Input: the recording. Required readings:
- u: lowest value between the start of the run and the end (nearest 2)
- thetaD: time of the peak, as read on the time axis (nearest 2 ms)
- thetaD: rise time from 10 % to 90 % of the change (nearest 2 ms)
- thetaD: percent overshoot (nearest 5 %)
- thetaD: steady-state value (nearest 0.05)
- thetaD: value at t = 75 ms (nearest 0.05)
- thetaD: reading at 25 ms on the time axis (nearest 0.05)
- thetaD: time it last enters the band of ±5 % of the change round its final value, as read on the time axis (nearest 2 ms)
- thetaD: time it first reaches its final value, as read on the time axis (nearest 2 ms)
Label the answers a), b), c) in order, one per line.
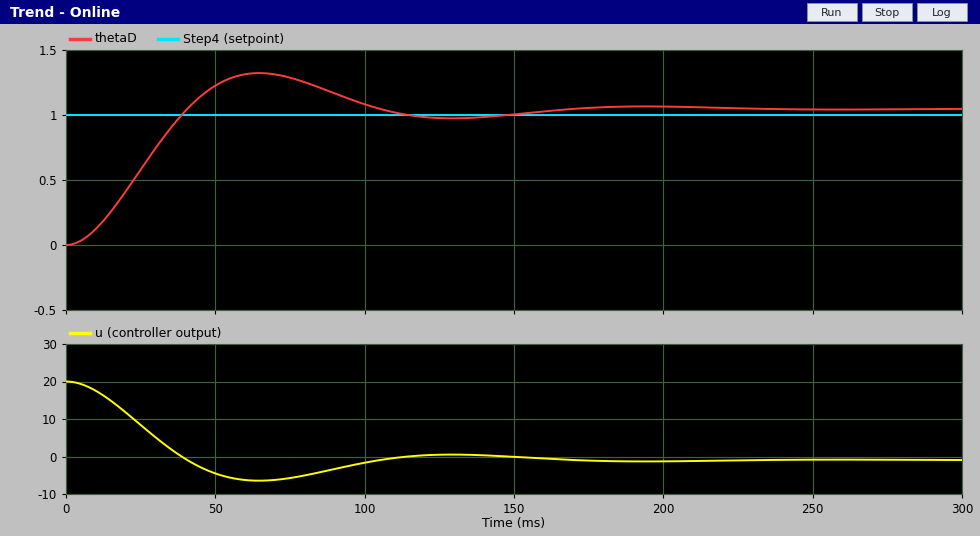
a) -6
b) 64 ms
c) 28 ms
d) 25 %
e) 1.05
f) 1.30
g) 0.60
h) 146 ms
i) 40 ms
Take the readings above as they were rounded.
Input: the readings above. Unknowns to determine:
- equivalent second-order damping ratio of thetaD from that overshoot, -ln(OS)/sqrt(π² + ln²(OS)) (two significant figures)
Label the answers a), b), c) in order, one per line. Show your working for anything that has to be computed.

a) ln(0.25) = -1.386; 1.386 / sqrt(9.870 + 1.922) = 0.40
